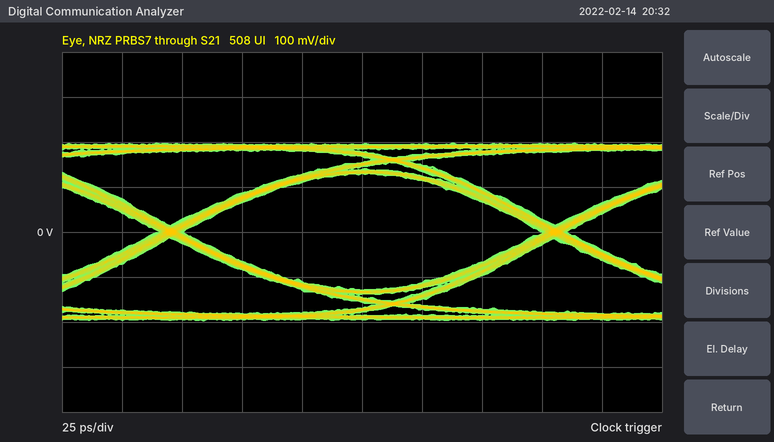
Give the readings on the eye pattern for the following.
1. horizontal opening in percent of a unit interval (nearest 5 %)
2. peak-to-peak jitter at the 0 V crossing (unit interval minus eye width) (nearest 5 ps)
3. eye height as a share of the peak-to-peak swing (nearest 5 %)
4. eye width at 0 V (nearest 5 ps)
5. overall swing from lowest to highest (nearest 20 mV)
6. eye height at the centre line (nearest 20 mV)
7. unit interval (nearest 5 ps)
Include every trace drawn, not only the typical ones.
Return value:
95 %
10 ps
65 %
150 ps
400 mV
260 mV
160 ps
